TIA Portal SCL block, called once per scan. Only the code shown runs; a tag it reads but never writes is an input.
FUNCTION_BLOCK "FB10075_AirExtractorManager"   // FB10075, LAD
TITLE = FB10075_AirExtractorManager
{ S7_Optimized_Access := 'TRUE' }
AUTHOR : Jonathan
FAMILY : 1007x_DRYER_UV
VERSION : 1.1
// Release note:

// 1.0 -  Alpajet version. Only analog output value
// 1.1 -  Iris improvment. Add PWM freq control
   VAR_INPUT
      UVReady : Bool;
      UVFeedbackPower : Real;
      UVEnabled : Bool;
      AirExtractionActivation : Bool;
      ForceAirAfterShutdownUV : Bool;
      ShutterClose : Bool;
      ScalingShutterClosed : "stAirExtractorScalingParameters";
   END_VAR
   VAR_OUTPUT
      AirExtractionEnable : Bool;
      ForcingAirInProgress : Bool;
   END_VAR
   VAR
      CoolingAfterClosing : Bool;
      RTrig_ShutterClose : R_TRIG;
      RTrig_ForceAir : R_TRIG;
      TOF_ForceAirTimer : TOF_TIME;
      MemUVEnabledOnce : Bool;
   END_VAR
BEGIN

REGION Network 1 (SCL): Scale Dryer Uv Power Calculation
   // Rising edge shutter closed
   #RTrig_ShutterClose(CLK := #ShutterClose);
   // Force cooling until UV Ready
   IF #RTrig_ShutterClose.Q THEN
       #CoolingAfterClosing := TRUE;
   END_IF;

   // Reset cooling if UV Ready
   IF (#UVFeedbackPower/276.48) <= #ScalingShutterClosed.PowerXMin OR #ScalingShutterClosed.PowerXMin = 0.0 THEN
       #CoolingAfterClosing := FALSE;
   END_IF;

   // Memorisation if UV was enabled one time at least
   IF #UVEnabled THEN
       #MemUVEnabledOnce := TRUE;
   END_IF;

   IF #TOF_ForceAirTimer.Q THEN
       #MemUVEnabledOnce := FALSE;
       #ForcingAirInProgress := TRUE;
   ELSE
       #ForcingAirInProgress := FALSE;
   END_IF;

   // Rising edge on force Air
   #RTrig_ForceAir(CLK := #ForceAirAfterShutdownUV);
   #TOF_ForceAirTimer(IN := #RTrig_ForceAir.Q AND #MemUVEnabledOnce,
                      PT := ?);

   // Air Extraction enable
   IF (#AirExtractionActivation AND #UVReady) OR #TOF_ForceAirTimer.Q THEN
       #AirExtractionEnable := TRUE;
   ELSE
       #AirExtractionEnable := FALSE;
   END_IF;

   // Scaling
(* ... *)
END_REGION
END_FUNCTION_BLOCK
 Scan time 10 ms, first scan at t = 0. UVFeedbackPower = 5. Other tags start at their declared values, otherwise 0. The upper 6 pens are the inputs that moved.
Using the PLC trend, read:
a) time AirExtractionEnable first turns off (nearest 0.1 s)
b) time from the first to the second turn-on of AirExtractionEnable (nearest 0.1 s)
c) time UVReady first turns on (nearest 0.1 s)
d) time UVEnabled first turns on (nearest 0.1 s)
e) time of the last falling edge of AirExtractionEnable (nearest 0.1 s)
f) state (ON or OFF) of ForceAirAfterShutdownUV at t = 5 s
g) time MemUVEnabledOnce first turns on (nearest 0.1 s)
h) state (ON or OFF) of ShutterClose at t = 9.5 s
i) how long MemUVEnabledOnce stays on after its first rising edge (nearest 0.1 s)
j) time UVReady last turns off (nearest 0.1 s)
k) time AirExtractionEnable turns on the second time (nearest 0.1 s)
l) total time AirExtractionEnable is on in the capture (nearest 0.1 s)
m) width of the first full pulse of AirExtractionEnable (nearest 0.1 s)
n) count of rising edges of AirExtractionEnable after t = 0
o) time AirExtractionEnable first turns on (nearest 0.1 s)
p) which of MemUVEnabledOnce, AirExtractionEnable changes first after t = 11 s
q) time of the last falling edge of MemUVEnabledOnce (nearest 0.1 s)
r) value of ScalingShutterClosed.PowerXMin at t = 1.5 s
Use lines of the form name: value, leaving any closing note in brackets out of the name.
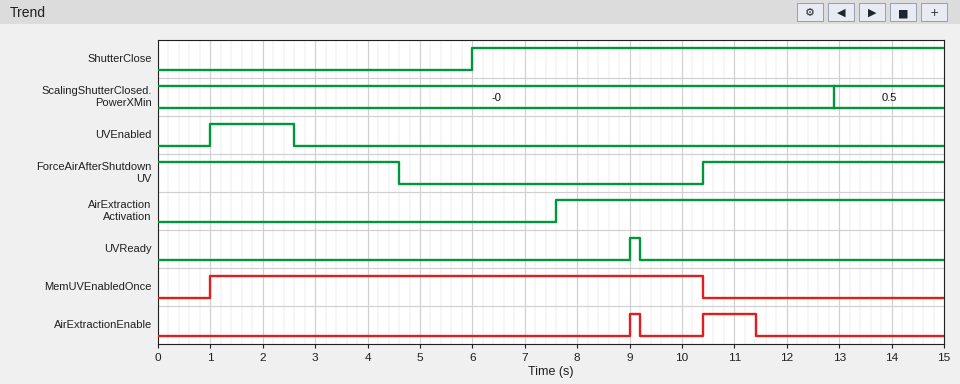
time AirExtractionEnable first turns off: 9.2 s
time from the first to the second turn-on of AirExtractionEnable: 1.4 s
time UVReady first turns on: 9.0 s
time UVEnabled first turns on: 1.0 s
time of the last falling edge of AirExtractionEnable: 11.4 s
state (ON or OFF) of ForceAirAfterShutdownUV at t = 5 s: OFF
time MemUVEnabledOnce first turns on: 1.0 s
state (ON or OFF) of ShutterClose at t = 9.5 s: ON
how long MemUVEnabledOnce stays on after its first rising edge: 9.4 s
time UVReady last turns off: 9.2 s
time AirExtractionEnable turns on the second time: 10.4 s
total time AirExtractionEnable is on in the capture: 1.2 s
width of the first full pulse of AirExtractionEnable: 0.2 s
count of rising edges of AirExtractionEnable after t = 0: 2
time AirExtractionEnable first turns on: 9.0 s
which of MemUVEnabledOnce, AirExtractionEnable changes first after t = 11 s: AirExtractionEnable
time of the last falling edge of MemUVEnabledOnce: 10.4 s
value of ScalingShutterClosed.PowerXMin at t = 1.5 s: -0
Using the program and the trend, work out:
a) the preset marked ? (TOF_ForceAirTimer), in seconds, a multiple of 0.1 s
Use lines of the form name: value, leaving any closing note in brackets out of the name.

the preset marked ? (TOF_ForceAirTimer), in seconds, a multiple of 0.1 s: 1.0 s
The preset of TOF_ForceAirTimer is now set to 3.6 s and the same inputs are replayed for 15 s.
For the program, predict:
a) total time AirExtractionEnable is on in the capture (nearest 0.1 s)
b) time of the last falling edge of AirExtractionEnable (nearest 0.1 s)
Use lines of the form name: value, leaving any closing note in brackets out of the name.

total time AirExtractionEnable is on in the capture: 3.8 s
time of the last falling edge of AirExtractionEnable: 14.0 s
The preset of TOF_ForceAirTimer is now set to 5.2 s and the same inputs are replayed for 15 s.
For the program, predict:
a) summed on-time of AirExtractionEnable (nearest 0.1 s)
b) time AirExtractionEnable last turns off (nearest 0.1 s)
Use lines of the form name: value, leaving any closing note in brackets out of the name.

summed on-time of AirExtractionEnable: 4.8 s
time AirExtractionEnable last turns off: 9.2 s
